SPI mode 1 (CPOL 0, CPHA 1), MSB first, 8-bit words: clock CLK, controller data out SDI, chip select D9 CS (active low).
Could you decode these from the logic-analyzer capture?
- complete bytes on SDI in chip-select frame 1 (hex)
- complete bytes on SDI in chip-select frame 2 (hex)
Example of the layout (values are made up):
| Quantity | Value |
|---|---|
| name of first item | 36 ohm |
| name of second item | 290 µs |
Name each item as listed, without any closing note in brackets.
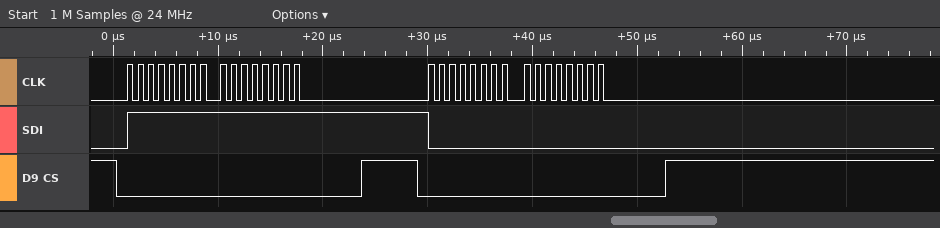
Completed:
| Quantity | Value |
|---|---|
| complete bytes on SDI in chip-select frame 1 | FF FF |
| complete bytes on SDI in chip-select frame 2 | 00 00 |
